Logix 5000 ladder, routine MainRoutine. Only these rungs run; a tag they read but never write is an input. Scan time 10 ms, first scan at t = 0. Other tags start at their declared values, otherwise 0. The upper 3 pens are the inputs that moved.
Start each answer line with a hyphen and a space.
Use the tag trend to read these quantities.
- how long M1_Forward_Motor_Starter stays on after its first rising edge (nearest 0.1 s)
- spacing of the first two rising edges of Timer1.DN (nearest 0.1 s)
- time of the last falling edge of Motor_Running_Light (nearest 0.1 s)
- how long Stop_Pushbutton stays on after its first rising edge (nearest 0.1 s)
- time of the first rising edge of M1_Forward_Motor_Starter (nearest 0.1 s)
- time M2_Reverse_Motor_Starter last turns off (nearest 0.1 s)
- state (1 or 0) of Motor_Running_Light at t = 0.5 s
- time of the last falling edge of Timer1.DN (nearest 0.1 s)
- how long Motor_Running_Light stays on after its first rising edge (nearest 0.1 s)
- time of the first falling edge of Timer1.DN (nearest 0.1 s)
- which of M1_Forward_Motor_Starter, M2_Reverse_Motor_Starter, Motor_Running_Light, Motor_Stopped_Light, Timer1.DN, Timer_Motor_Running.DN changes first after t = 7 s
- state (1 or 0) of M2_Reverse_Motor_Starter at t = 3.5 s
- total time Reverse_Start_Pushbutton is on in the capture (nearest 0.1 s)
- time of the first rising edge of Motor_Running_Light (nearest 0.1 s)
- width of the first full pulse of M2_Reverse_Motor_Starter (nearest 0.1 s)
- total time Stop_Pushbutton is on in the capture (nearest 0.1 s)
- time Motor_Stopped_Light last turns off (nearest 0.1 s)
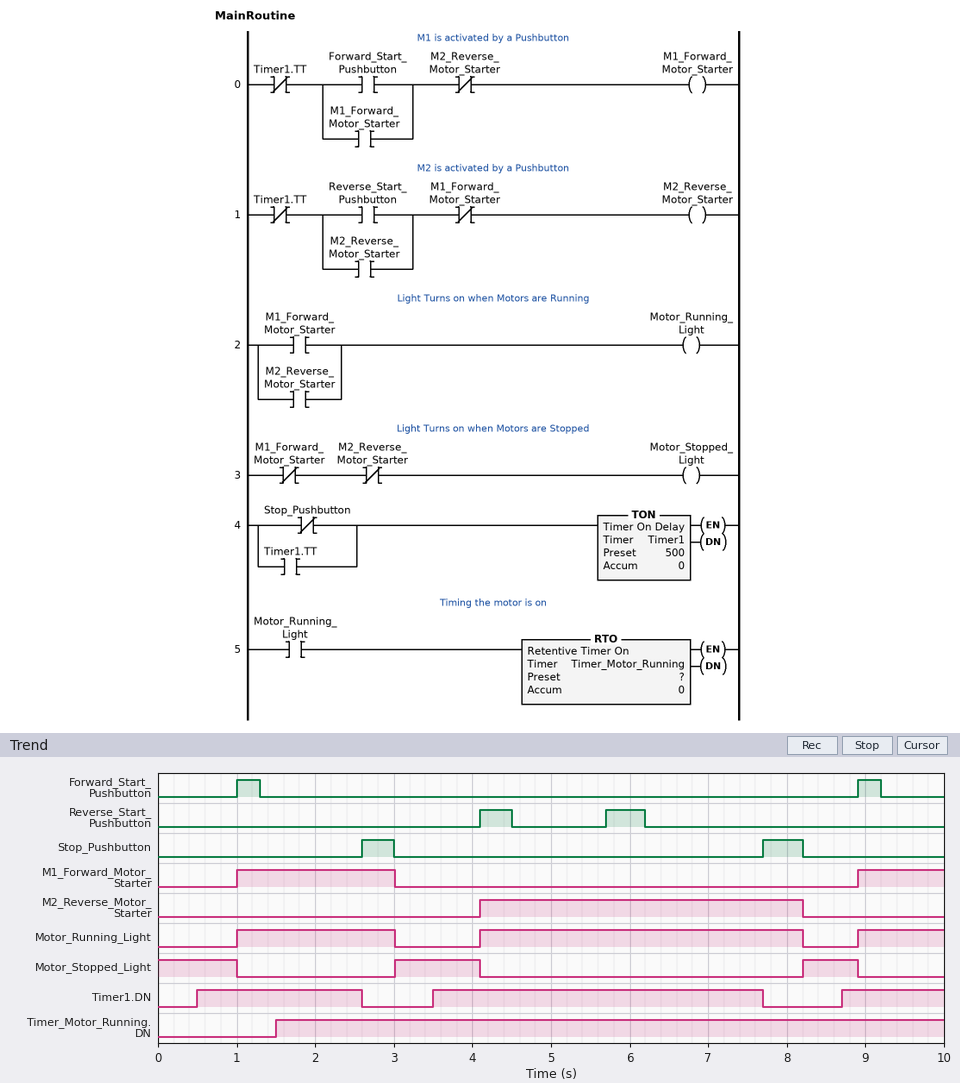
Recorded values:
- 2.0 s
- 3.0 s
- 8.2 s
- 0.4 s
- 1.0 s
- 8.2 s
- 0
- 7.7 s
- 2.0 s
- 2.6 s
- Timer1.DN
- 0
- 0.9 s
- 1.0 s
- 4.1 s
- 0.9 s
- 8.9 s
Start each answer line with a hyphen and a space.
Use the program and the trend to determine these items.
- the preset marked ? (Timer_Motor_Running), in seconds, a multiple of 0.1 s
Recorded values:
- 0.5 s
